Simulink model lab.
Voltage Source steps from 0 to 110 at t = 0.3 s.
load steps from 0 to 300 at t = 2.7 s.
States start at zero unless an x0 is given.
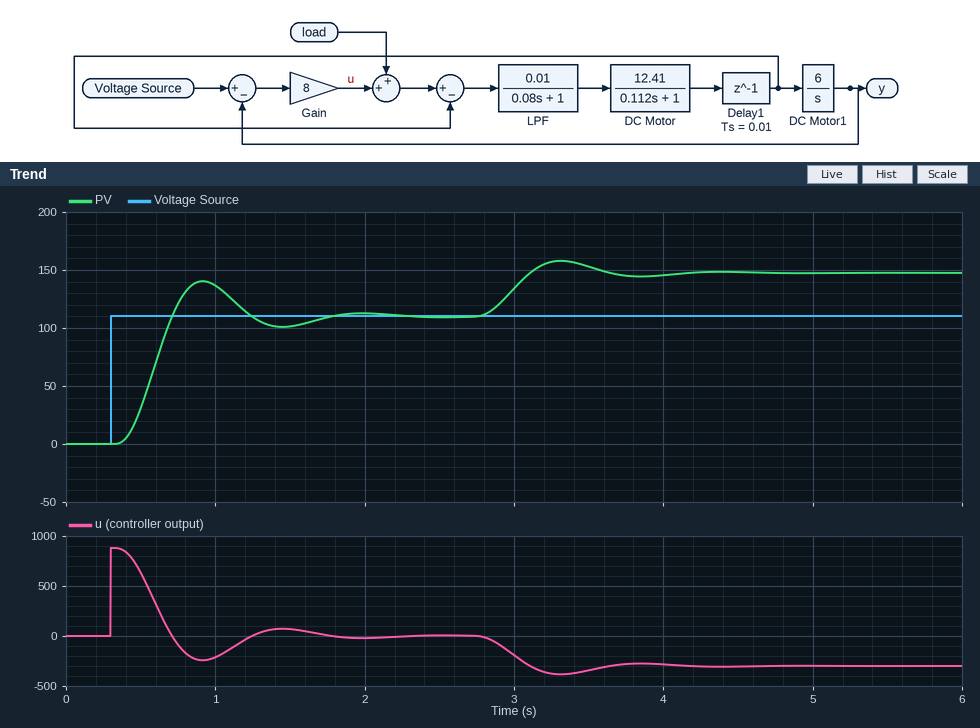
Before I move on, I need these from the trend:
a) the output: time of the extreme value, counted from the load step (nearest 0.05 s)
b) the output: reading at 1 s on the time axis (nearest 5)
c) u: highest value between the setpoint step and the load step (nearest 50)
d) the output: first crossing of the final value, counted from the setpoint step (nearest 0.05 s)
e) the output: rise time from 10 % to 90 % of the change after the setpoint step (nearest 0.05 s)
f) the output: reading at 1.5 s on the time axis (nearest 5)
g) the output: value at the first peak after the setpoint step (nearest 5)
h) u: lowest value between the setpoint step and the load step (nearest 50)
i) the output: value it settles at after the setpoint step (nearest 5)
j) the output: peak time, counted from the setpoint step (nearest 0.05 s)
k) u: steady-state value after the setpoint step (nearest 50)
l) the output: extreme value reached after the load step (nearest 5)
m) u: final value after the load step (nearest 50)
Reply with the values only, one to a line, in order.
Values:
0.60 s
135
900
0.40 s
0.25 s
100
140
-250
110
0.60 s
0
160
-300
